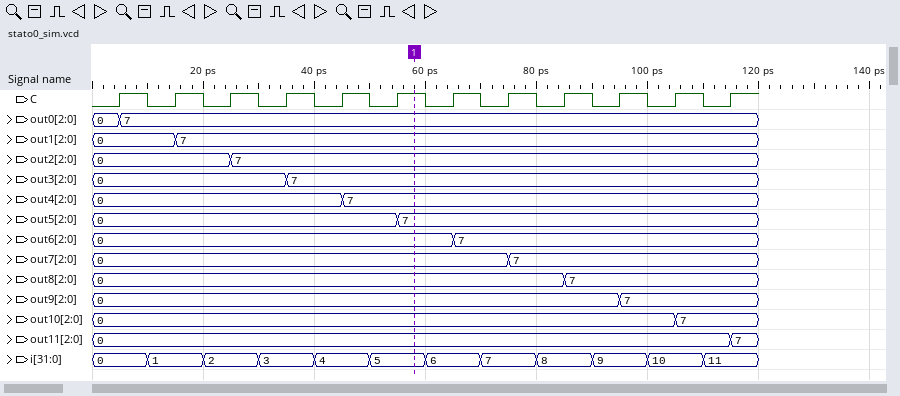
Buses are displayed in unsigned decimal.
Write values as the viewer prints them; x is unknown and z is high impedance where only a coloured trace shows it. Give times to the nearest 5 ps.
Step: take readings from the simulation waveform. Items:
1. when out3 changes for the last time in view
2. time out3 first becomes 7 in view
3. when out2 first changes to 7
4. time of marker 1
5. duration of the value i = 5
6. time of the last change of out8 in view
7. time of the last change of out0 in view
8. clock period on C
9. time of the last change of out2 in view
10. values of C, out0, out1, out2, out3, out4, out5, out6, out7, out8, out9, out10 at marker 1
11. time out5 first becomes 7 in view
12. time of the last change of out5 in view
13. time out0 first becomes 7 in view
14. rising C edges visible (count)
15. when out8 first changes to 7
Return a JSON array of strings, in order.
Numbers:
["35 ps", "35 ps", "25 ps", "60 ps", "10 ps", "85 ps", "5 ps", "10 ps", "25 ps", "C=1, out0=7, out1=7, out2=7, out3=7, out4=7, out5=7, out6=0, out7=0, out8=0, out9=0, out10=0", "55 ps", "55 ps", "5 ps", "12", "85 ps"]
